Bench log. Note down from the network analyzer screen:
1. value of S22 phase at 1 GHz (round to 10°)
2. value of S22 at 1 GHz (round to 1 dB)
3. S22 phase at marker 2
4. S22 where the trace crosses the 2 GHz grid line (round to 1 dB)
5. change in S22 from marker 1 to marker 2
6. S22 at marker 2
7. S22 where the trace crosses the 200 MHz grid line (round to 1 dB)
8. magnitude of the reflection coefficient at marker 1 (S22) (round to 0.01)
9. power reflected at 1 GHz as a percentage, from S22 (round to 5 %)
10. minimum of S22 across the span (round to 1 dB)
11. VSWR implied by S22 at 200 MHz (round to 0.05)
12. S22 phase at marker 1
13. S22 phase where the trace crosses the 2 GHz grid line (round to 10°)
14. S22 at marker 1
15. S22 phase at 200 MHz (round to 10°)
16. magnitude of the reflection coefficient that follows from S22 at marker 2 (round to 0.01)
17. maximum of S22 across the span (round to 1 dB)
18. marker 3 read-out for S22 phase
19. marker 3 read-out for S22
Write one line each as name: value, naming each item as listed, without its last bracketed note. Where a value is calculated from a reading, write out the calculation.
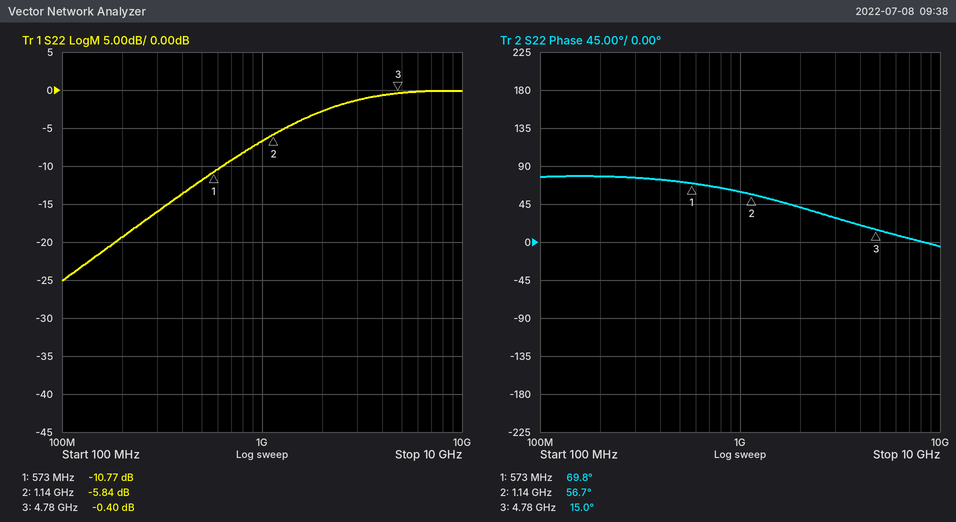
value of S22 phase at 1 GHz: 60°
value of S22 at 1 GHz: -7 dB
S22 phase at marker 2: 56.7°
S22 where the trace crosses the 2 GHz grid line: -3 dB
change in S22 from marker 1 to marker 2: -5.84 − (-10.77) = 4.93 dB
S22 at marker 2: -5.84 dB
S22 where the trace crosses the 200 MHz grid line: -19 dB
magnitude of the reflection coefficient at marker 1 (S22): 10^(-10.77/20) ≈ 0.29
power reflected at 1 GHz as a percentage, from S22: 10^(-7/10) ≈ 20 %
minimum of S22 across the span: -25 dB
VSWR implied by S22 at 200 MHz: |Γ| = 10^(-19/20) = 0.1122; VSWR = (1 + 0.1122)/(1 − 0.1122) ≈ 1.25
S22 phase at marker 1: 69.8°
S22 phase where the trace crosses the 2 GHz grid line: 40°
S22 at marker 1: -10.77 dB
S22 phase at 200 MHz: 80°
magnitude of the reflection coefficient that follows from S22 at marker 2: 10^(-5.84/20) ≈ 0.51
maximum of S22 across the span: 0 dB
marker 3 read-out for S22 phase: 15.0°
marker 3 read-out for S22: -0.40 dB
